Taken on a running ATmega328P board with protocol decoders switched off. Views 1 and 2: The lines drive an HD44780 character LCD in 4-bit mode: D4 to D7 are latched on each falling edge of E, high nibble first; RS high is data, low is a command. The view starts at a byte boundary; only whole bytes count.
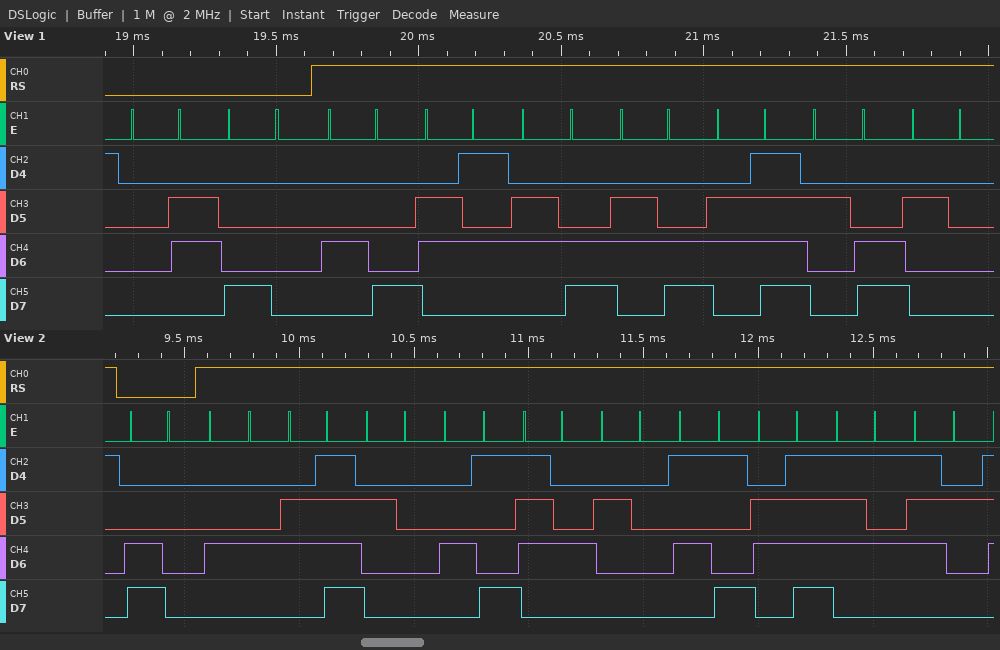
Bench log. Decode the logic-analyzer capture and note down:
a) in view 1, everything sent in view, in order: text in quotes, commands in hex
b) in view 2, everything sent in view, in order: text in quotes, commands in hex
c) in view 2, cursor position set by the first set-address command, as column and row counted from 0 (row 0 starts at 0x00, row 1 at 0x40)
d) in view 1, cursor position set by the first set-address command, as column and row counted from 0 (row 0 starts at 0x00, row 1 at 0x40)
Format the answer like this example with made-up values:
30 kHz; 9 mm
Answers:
0x06 0x80 "Hello, "; 0xC0 "Do It Your"; column 0, row 1; column 0, row 0
